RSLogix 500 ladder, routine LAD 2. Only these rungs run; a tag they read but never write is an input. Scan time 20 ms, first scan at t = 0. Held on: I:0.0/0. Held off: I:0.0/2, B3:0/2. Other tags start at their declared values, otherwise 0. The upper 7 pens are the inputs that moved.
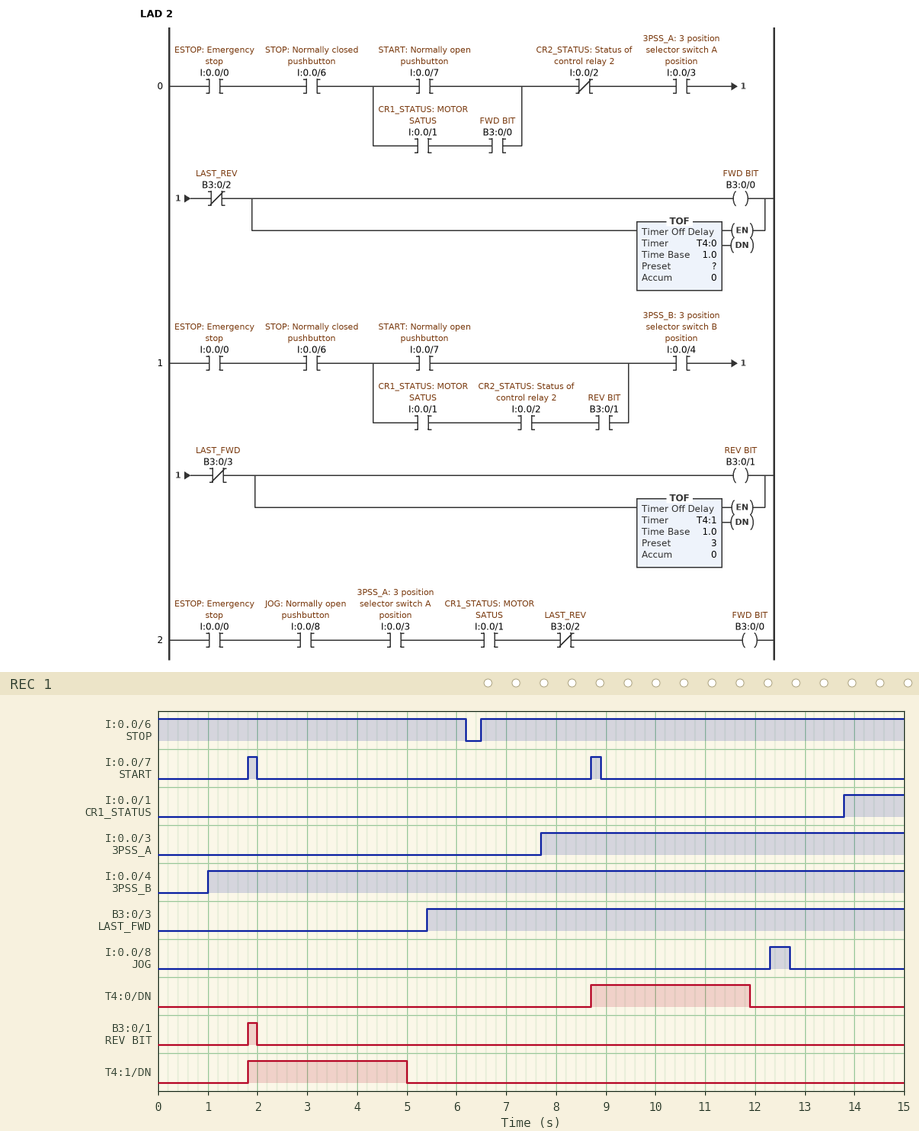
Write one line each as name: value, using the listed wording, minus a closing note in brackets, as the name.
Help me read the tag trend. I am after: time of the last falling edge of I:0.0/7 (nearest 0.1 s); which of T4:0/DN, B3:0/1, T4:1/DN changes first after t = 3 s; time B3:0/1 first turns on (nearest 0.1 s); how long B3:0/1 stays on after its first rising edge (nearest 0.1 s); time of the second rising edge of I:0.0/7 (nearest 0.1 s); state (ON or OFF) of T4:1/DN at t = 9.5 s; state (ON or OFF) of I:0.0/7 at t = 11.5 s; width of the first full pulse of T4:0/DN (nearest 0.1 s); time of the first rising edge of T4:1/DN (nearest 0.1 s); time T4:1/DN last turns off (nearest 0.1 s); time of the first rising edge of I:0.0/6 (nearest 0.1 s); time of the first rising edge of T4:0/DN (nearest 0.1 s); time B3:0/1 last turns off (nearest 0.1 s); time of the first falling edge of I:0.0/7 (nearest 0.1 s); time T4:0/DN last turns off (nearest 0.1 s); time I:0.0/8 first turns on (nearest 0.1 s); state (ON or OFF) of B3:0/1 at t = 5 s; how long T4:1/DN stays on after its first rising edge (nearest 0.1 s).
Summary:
time of the last falling edge of I:0.0/7: 8.9 s
which of T4:0/DN, B3:0/1, T4:1/DN changes first after t = 3 s: T4:1/DN
time B3:0/1 first turns on: 1.8 s
how long B3:0/1 stays on after its first rising edge: 0.2 s
time of the second rising edge of I:0.0/7: 8.7 s
state (ON or OFF) of T4:1/DN at t = 9.5 s: OFF
state (ON or OFF) of I:0.0/7 at t = 11.5 s: OFF
width of the first full pulse of T4:0/DN: 3.2 s
time of the first rising edge of T4:1/DN: 1.8 s
time T4:1/DN last turns off: 5.0 s
time of the first rising edge of I:0.0/6: 6.5 s
time of the first rising edge of T4:0/DN: 8.7 s
time B3:0/1 last turns off: 2.0 s
time of the first falling edge of I:0.0/7: 2.0 s
time T4:0/DN last turns off: 11.9 s
time I:0.0/8 first turns on: 12.3 s
state (ON or OFF) of B3:0/1 at t = 5 s: OFF
how long T4:1/DN stays on after its first rising edge: 3.2 s
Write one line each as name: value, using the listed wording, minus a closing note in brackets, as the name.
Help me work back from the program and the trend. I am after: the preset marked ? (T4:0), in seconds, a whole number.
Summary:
the preset marked ? (T4:0), in seconds, a whole number: 3 s
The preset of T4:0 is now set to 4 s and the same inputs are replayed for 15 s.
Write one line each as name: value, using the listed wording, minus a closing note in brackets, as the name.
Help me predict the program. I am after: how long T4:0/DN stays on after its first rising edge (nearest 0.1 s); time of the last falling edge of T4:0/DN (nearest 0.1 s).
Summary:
how long T4:0/DN stays on after its first rising edge: 4.2 s
time of the last falling edge of T4:0/DN: 12.9 s
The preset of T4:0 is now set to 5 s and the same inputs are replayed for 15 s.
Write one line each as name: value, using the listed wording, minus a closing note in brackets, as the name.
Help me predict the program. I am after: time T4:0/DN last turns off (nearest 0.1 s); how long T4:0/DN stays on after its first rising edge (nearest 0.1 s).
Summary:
time T4:0/DN last turns off: 13.9 s
how long T4:0/DN stays on after its first rising edge: 5.2 s
